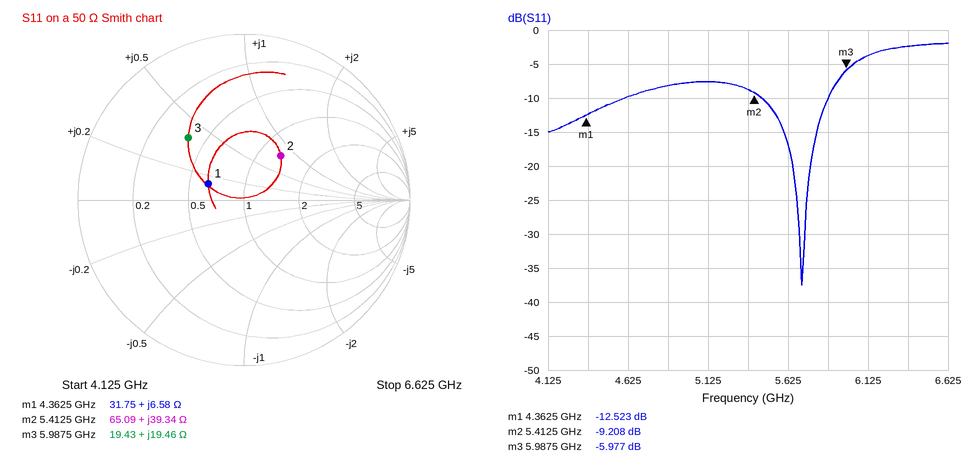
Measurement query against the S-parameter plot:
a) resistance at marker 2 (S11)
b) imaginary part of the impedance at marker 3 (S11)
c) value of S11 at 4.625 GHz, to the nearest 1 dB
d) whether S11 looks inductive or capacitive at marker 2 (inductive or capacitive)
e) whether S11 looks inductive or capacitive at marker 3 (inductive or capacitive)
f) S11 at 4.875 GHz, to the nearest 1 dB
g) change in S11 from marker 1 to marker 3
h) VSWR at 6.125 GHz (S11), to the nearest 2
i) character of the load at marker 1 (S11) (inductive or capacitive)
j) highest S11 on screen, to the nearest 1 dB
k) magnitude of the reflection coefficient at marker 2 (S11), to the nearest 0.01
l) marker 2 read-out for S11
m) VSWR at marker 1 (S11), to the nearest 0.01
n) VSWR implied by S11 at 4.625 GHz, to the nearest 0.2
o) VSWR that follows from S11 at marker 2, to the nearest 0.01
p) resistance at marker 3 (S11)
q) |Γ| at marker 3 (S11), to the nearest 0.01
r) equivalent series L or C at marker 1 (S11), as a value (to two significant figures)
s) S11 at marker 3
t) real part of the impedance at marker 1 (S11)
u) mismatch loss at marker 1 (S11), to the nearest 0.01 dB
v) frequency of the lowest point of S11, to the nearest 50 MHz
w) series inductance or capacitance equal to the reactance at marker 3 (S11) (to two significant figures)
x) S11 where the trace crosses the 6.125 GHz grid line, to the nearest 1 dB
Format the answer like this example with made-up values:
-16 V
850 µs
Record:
65.09 Ω
+19.46 Ω
-10 dB
inductive
inductive
-8 dB
6.546 dB
4
inductive
-2 dB
0.35
-9.208 dB
1.62
2.0
2.06
19.43 Ω
0.50
240 pH
-5.977 dB
31.75 Ω
0.25 dB
5.70 GHz
520 pH
-4 dB
